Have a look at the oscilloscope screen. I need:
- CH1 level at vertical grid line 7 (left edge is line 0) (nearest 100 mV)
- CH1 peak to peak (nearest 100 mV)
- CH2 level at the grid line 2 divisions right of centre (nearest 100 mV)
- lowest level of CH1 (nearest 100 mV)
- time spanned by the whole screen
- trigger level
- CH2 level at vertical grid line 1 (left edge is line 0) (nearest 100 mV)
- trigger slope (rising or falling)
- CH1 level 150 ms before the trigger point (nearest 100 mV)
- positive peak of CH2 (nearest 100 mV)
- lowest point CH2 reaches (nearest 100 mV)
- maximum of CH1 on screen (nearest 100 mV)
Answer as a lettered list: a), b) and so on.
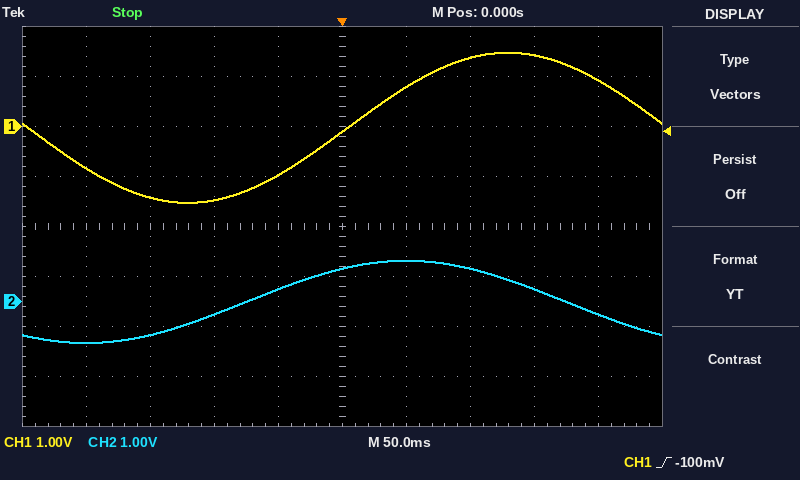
a) 1.4 V
b) 3.0 V
c) 700 mV
d) -1.5 V
e) 500 ms
f) -100 mV
g) -800 mV
h) rising
i) -1.4 V
j) 800 mV
k) -800 mV
l) 1.5 V
